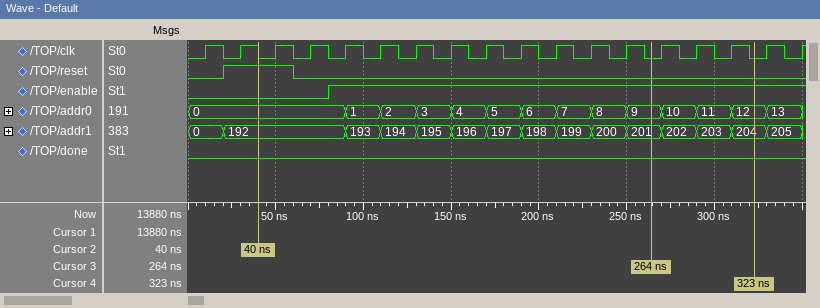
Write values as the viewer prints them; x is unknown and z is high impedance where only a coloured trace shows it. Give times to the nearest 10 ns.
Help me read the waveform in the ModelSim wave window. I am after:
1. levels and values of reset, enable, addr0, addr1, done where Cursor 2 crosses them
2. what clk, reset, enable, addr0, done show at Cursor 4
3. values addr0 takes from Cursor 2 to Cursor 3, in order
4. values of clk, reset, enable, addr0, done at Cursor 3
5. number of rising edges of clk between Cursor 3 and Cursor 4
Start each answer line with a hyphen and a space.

- reset=1, enable=0, addr0=0, addr1=192, done=0
- clk=0, reset=0, enable=1, addr0=12, done=0
- 0, 1, 2, 3, 4, 5, 6, 7, 8, 9
- clk=0, reset=0, enable=1, addr0=9, done=0
- 3
